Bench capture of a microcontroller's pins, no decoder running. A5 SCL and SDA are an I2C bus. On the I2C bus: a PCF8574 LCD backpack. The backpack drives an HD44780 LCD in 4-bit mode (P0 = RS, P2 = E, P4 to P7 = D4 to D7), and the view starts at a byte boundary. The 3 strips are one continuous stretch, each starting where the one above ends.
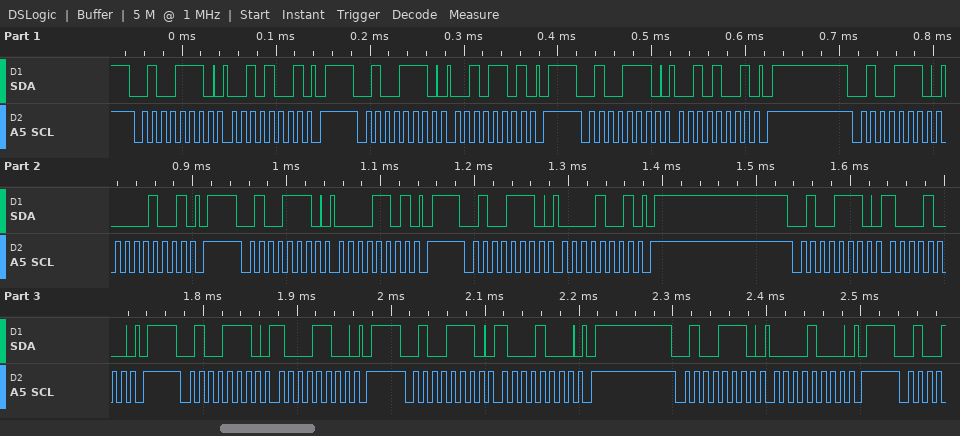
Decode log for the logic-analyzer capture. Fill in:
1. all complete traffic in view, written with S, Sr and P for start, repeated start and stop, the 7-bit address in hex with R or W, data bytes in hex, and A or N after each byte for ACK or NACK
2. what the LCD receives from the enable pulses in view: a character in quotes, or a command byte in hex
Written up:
S 27W A 29 A P S 27W A 2D A P S 27W A 29 A P S 27W A 09 A P S 27W A 0D A P S 27W A 09 A P S 27W A 88 A P S 27W A 8C A P S 27W A 88 A P S 27W A 08 A P
' '
